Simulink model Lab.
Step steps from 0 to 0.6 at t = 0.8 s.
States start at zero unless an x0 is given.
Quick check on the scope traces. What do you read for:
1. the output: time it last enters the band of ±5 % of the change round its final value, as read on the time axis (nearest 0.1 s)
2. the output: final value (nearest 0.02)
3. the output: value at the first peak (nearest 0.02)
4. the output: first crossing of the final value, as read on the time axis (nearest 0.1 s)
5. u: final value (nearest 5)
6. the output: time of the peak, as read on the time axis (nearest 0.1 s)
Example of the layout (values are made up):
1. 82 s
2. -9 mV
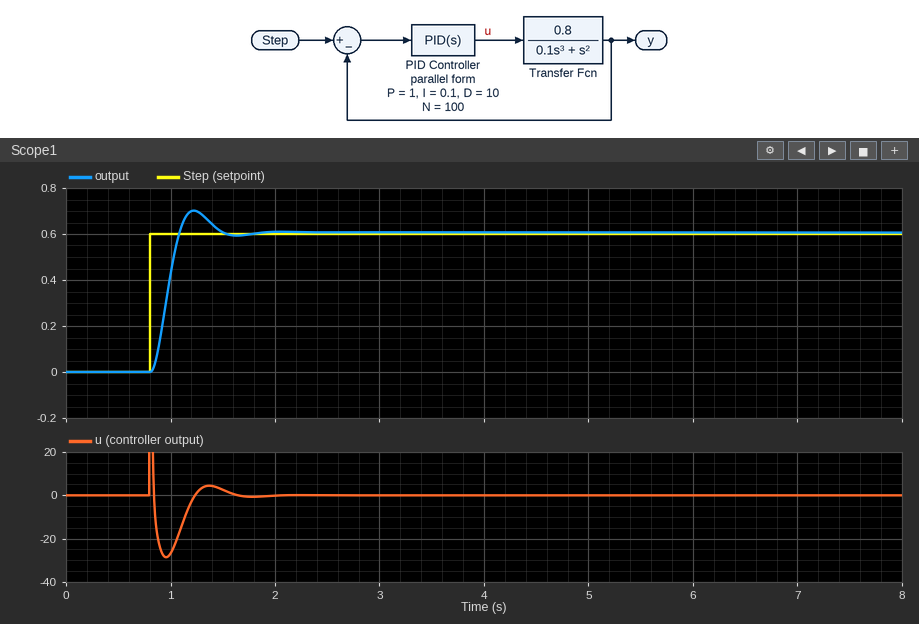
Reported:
1. 1.4 s
2. 0.60
3. 0.70
4. 1.1 s
5. 0
6. 1.2 s
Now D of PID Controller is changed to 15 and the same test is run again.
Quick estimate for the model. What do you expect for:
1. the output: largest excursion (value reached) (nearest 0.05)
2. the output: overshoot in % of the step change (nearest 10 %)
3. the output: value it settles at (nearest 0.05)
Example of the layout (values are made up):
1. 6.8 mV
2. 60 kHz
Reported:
1. 0.75
2. 30 %
3. 0.60
